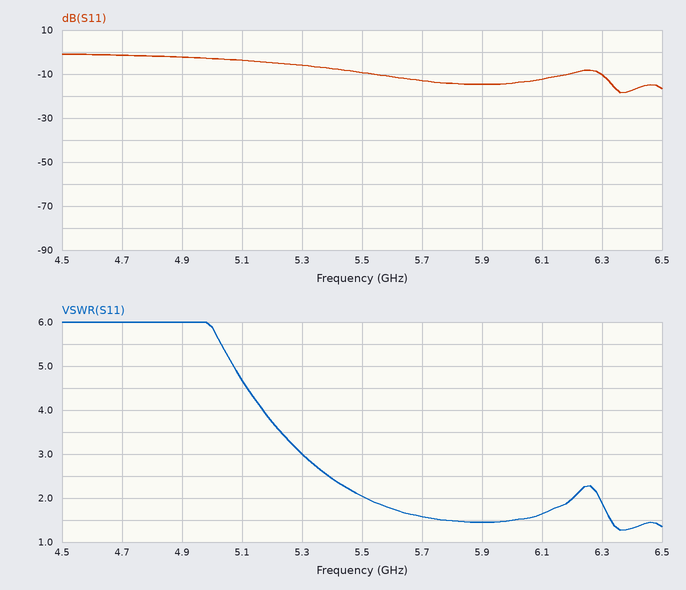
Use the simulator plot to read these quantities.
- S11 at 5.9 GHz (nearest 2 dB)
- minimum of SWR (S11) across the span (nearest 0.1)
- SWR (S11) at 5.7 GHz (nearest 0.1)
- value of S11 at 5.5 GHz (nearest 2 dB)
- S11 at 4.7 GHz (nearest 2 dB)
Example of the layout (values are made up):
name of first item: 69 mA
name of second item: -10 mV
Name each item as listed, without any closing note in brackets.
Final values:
S11 at 5.9 GHz: -14 dB
minimum of SWR (S11) across the span: 1.3
SWR (S11) at 5.7 GHz: 1.6
value of S11 at 5.5 GHz: -10 dB
S11 at 4.7 GHz: -2 dB
